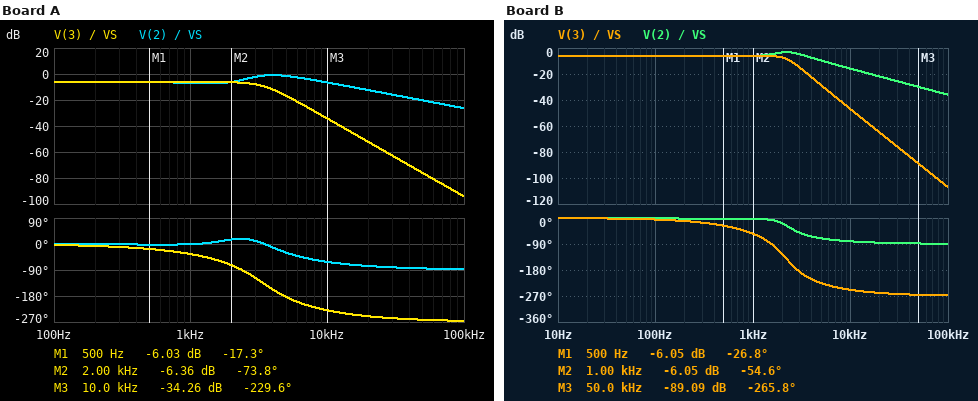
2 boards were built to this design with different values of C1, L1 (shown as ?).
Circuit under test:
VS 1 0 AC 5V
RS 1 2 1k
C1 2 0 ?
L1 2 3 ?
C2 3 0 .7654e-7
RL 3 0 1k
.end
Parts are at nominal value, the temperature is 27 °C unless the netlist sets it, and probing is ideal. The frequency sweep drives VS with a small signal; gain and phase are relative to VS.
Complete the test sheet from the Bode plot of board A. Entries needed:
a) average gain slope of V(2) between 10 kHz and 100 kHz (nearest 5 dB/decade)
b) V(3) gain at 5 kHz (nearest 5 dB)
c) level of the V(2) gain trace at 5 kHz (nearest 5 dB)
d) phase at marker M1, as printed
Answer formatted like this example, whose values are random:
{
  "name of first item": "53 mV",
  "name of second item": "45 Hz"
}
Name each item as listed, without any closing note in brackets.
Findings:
{
  "average gain slope of V(2) between 10 kHz and 100 kHz": "-20 dB/decade",
  "V(3) gain at 5 kHz": "-15 dB",
  "level of the V(2) gain trace at 5 kHz": "0 dB",
  "phase at marker M1, as printed": "-17.3 deg"
}
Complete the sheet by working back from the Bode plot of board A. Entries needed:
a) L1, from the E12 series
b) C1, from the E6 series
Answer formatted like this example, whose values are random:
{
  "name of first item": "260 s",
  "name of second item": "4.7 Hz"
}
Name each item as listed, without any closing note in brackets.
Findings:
{
  "L1, from the E12 series": "82 mH",
  "C1, from the E6 series": "33 nF"
}
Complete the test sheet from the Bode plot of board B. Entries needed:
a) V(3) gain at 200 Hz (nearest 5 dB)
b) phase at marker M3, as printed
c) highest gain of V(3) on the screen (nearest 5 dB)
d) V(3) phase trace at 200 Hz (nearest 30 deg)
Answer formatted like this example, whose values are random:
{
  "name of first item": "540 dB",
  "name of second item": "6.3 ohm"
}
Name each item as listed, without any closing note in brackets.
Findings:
{
  "V(3) gain at 200 Hz": "-5 dB",
  "phase at marker M3, as printed": "-265.8 deg",
  "highest gain of V(3) on the screen": "-5 dB",
  "V(3) phase trace at 200 Hz": "0 deg"
}
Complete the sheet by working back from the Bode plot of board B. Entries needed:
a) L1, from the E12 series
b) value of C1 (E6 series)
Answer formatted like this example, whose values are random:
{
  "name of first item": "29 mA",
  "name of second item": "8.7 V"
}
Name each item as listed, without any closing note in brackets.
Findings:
{
  "L1, from the E12 series": "120 mH",
  "value of C1": "100 nF"
}
